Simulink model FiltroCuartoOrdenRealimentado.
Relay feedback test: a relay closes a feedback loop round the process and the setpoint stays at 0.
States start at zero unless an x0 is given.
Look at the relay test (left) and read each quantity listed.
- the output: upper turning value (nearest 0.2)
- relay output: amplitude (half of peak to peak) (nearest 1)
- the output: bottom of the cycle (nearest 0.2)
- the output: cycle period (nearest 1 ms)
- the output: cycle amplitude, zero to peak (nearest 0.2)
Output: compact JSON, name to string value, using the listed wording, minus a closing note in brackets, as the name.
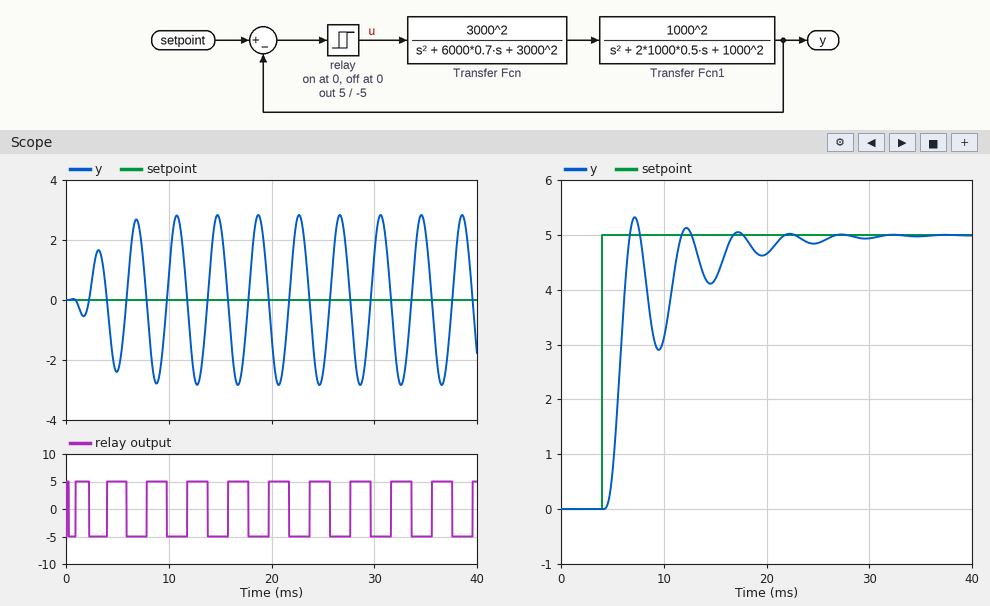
{"the output: upper turning value": "2.8", "relay output: amplitude (half of peak to peak)": "5", "the output: bottom of the cycle": "-2.8", "the output: cycle period": "4 ms", "the output: cycle amplitude, zero to peak": "2.8"}
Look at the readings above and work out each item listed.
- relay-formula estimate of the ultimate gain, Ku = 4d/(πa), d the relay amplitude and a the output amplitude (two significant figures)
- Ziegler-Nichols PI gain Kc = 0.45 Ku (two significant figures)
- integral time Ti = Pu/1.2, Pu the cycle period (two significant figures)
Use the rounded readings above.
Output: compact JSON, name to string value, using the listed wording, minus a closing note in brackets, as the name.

{"relay-formula estimate of the ultimate gain, Ku = 4d/(πa), d the relay amplitude and a the output amplitude": "2.3", "Ziegler-Nichols PI gain Kc = 0.45 Ku": "1.0", "integral time Ti = Pu/1.2, Pu the cycle period": "3.3 ms"}
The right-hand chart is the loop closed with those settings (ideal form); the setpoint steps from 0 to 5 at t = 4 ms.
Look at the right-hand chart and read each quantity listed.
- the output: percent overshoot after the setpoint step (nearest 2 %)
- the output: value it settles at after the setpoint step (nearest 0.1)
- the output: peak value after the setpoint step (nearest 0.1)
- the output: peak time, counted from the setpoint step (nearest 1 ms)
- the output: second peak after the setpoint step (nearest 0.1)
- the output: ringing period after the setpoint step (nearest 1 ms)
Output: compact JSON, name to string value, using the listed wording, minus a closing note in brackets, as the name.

{"the output: percent overshoot after the setpoint step": "6 %", "the output: value it settles at after the setpoint step": "5.0", "the output: peak value after the setpoint step": "5.3", "the output: peak time, counted from the setpoint step": "3 ms", "the output: second peak after the setpoint step": "5.1", "the output: ringing period after the setpoint step": "5 ms"}
